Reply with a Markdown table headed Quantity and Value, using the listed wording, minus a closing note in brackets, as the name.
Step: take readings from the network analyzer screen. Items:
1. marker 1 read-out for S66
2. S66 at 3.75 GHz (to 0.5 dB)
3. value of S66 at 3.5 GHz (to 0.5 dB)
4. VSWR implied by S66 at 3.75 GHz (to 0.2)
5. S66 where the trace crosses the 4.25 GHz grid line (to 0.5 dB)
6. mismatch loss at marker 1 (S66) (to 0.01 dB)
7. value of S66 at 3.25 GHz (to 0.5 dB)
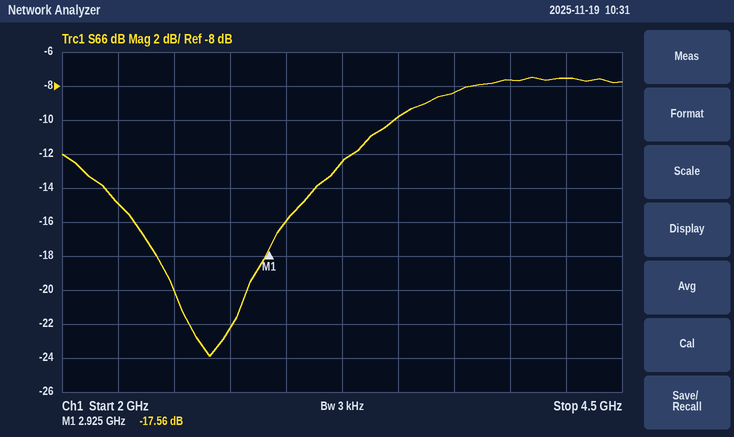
| Quantity | Value |
|---|---|
| marker 1 read-out for S66 | -17.56 dB |
| S66 at 3.75 GHz | -8.5 dB |
| value of S66 at 3.5 GHz | -10.0 dB |
| VSWR implied by S66 at 3.75 GHz | 2.2 |
| S66 where the trace crosses the 4.25 GHz grid line | -7.5 dB |
| mismatch loss at marker 1 (S66) | 0.08 dB |
| value of S66 at 3.25 GHz | -12.5 dB |
